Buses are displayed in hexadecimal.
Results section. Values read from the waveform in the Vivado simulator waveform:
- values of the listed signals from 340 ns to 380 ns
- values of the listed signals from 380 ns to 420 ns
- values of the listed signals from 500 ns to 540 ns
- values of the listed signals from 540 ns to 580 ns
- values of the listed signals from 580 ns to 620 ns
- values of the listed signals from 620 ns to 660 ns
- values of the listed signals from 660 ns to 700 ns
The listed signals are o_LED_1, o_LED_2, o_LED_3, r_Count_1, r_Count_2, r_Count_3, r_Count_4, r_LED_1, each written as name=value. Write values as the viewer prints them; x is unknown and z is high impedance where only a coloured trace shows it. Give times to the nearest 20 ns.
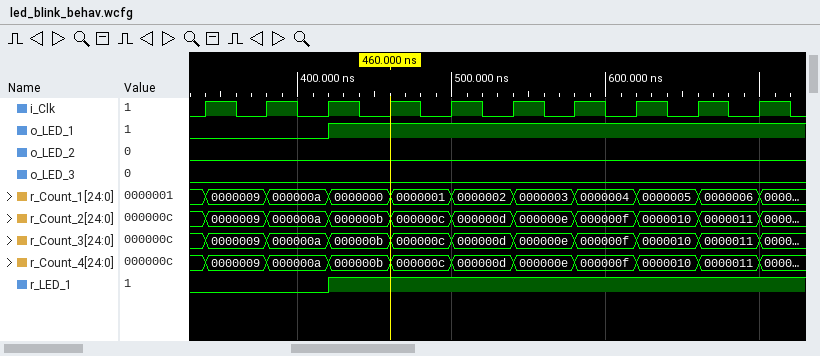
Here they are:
o_LED_1=0, o_LED_2=0, o_LED_3=0, r_Count_1=0000009, r_Count_2=0000009, r_Count_3=0000009, r_Count_4=0000009, r_LED_1=0
o_LED_1=0, o_LED_2=0, o_LED_3=0, r_Count_1=000000a, r_Count_2=000000a, r_Count_3=000000a, r_Count_4=000000a, r_LED_1=0
o_LED_1=1, o_LED_2=0, o_LED_3=0, r_Count_1=0000002, r_Count_2=000000d, r_Count_3=000000d, r_Count_4=000000d, r_LED_1=1
o_LED_1=1, o_LED_2=0, o_LED_3=0, r_Count_1=0000003, r_Count_2=000000e, r_Count_3=000000e, r_Count_4=000000e, r_LED_1=1
o_LED_1=1, o_LED_2=0, o_LED_3=0, r_Count_1=0000004, r_Count_2=000000f, r_Count_3=000000f, r_Count_4=000000f, r_LED_1=1
o_LED_1=1, o_LED_2=0, o_LED_3=0, r_Count_1=0000005, r_Count_2=0000010, r_Count_3=0000010, r_Count_4=0000010, r_LED_1=1
o_LED_1=1, o_LED_2=0, o_LED_3=0, r_Count_1=0000006, r_Count_2=0000011, r_Count_3=0000011, r_Count_4=0000011, r_LED_1=1
